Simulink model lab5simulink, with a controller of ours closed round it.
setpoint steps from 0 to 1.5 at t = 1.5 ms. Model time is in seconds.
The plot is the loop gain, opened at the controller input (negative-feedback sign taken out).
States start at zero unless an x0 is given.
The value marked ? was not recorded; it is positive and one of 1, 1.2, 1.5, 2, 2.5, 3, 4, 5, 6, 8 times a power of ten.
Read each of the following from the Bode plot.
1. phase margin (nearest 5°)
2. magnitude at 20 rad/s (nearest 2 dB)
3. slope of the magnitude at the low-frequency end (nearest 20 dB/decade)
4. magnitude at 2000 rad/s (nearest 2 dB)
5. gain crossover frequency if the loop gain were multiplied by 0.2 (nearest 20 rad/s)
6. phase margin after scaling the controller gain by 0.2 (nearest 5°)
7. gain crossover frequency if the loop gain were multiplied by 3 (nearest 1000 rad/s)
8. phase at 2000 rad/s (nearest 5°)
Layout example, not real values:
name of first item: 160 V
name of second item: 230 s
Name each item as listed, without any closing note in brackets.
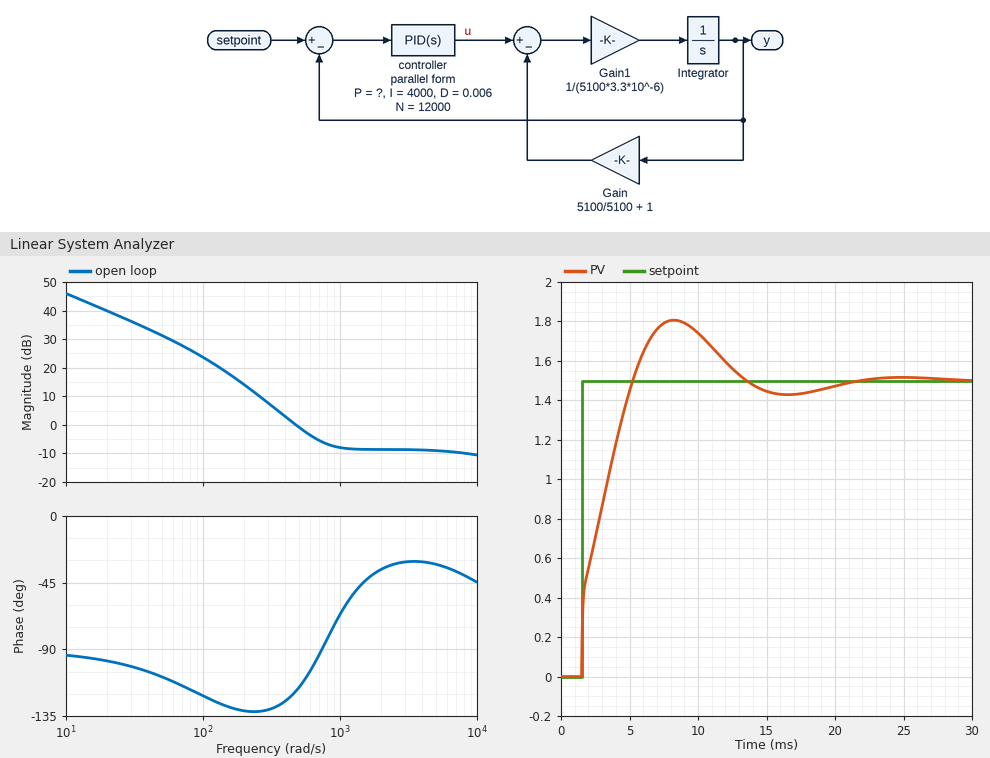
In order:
phase margin: 60°
magnitude at 20 rad/s: 40 dB
slope of the magnitude at the low-frequency end: -20 dB/decade
magnitude at 2000 rad/s: -8 dB
gain crossover frequency if the loop gain were multiplied by 0.2: 200 rad/s
phase margin after scaling the controller gain by 0.2: 50°
gain crossover frequency if the loop gain were multiplied by 3: 7000 rad/s
phase at 2000 rad/s: -35°
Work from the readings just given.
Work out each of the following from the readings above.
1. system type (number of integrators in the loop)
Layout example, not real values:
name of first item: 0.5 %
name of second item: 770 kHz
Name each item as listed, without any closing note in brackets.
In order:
system type: 1
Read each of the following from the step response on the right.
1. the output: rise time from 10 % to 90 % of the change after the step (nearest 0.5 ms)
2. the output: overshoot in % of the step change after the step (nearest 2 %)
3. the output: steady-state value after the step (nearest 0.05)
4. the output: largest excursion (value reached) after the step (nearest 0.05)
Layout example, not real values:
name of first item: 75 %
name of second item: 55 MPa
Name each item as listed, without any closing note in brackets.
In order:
the output: rise time from 10 % to 90 % of the change after the step: 3.0 ms
the output: overshoot in % of the step change after the step: 20 %
the output: steady-state value after the step: 1.50
the output: largest excursion (value reached) after the step: 1.80
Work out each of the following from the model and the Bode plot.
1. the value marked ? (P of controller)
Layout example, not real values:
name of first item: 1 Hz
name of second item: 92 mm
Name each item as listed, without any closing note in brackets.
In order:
the value marked ?: 6
